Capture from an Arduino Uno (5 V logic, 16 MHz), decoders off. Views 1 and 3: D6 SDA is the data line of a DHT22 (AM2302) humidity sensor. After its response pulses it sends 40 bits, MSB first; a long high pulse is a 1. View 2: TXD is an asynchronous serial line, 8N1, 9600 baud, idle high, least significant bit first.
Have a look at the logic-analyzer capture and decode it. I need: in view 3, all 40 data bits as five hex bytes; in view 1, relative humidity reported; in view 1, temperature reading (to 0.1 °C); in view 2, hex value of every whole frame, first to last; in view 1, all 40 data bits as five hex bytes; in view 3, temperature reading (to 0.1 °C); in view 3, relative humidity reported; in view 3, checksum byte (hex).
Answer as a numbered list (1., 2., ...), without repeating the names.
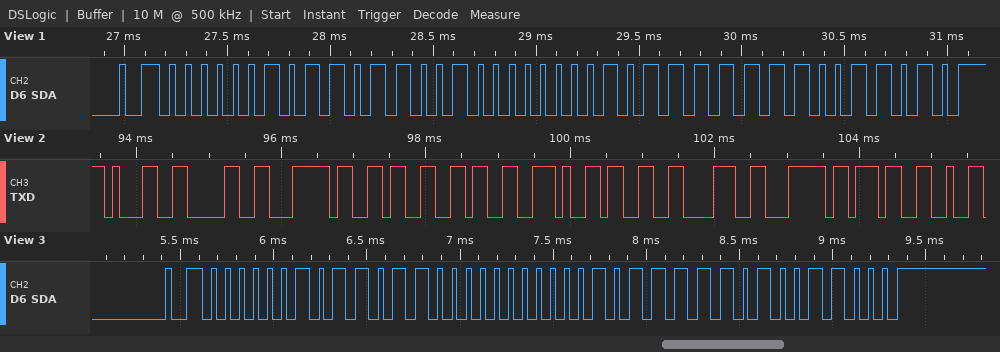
1. 02 D8 00 BE 98
2. 72.9 %
3. 19.1 °C
4. 0x31 0x30 0x7C 0x36 0x36 0x2E 0x33 0x38 0x7C 0x37
5. 02 D9 00 BF 9A
6. 19.0 °C
7. 72.8 %
8. 0x98
